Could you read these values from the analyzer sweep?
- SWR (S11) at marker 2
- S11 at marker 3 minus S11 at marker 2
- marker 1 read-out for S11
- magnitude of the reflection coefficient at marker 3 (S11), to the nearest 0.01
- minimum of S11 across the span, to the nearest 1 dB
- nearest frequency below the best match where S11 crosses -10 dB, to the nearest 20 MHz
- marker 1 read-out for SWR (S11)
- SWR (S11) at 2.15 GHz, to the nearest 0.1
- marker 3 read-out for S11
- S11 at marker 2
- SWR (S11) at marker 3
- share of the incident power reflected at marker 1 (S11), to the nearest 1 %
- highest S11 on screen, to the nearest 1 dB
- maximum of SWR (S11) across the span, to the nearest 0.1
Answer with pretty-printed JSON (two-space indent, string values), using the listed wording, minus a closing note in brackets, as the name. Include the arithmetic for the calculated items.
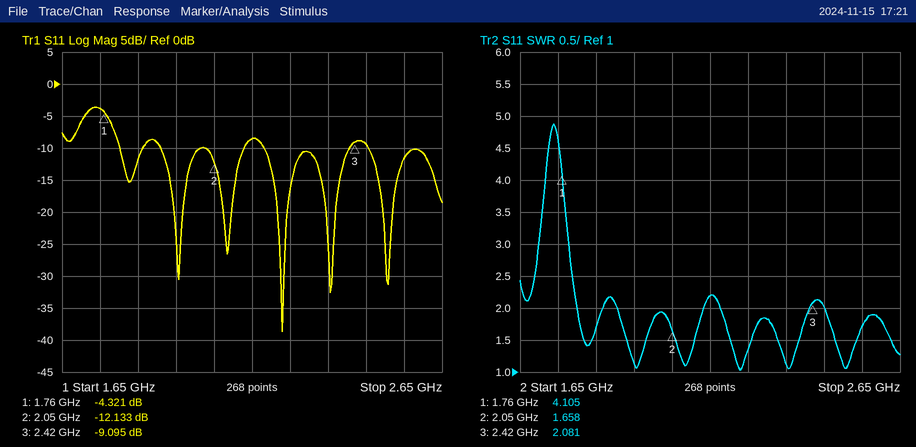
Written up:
{
  "SWR (S11) at marker 2": "1.658",
  "S11 at marker 3 minus S11 at marker 2": "-9.095 − (-12.133) = 3.038 dB",
  "marker 1 read-out for S11": "-4.321 dB",
  "magnitude of the reflection coefficient at marker 3 (S11), to the nearest 0.01": "10^(-9.095/20) ≈ 0.35",
  "minimum of S11 across the span, to the nearest 1 dB": "-39 dB",
  "nearest frequency below the best match where S11 crosses -10 dB, to the nearest 20 MHz": "2.18 GHz",
  "marker 1 read-out for SWR": "4.105",
  "SWR (S11) at 2.15 GHz, to the nearest 0.1": "2.2",
  "marker 3 read-out for S11": "-9.095 dB",
  "S11 at marker 2": "-12.133 dB",
  "SWR (S11) at marker 3": "2.081",
  "share of the incident power reflected at marker 1 (S11), to the nearest 1 %": "10^(-4.321/10) ≈ 37 %",
  "highest S11 on screen, to the nearest 1 dB": "-4 dB",
  "maximum of SWR (S11) across the span, to the nearest 0.1": "4.9"
}
